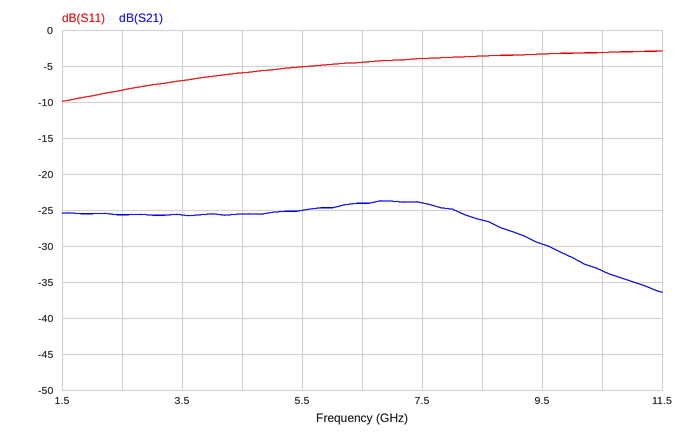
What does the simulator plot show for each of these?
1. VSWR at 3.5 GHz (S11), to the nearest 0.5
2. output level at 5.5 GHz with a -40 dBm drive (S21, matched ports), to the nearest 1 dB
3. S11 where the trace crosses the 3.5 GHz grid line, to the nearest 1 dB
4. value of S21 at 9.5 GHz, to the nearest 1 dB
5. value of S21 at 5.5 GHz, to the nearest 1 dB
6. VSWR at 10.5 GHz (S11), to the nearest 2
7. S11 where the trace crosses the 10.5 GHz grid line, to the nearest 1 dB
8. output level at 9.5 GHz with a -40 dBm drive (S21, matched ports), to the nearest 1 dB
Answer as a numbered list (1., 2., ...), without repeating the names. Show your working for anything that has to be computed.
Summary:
1. |Γ| = 10^(-7/20) = 0.4467; VSWR = (1 + 0.4467)/(1 − 0.4467) ≈ 2.61, so 2.5 to the nearest 0.5
2. -40 dBm + (-25 dB) = -65 dBm
3. -7 dB
4. -30 dB
5. -25 dB
6. |Γ| = 10^(-3/20) = 0.7079; VSWR = (1 + 0.7079)/(1 − 0.7079) ≈ 6
7. -3 dB
8. -40 dBm + (-30 dB) = -70 dBm
